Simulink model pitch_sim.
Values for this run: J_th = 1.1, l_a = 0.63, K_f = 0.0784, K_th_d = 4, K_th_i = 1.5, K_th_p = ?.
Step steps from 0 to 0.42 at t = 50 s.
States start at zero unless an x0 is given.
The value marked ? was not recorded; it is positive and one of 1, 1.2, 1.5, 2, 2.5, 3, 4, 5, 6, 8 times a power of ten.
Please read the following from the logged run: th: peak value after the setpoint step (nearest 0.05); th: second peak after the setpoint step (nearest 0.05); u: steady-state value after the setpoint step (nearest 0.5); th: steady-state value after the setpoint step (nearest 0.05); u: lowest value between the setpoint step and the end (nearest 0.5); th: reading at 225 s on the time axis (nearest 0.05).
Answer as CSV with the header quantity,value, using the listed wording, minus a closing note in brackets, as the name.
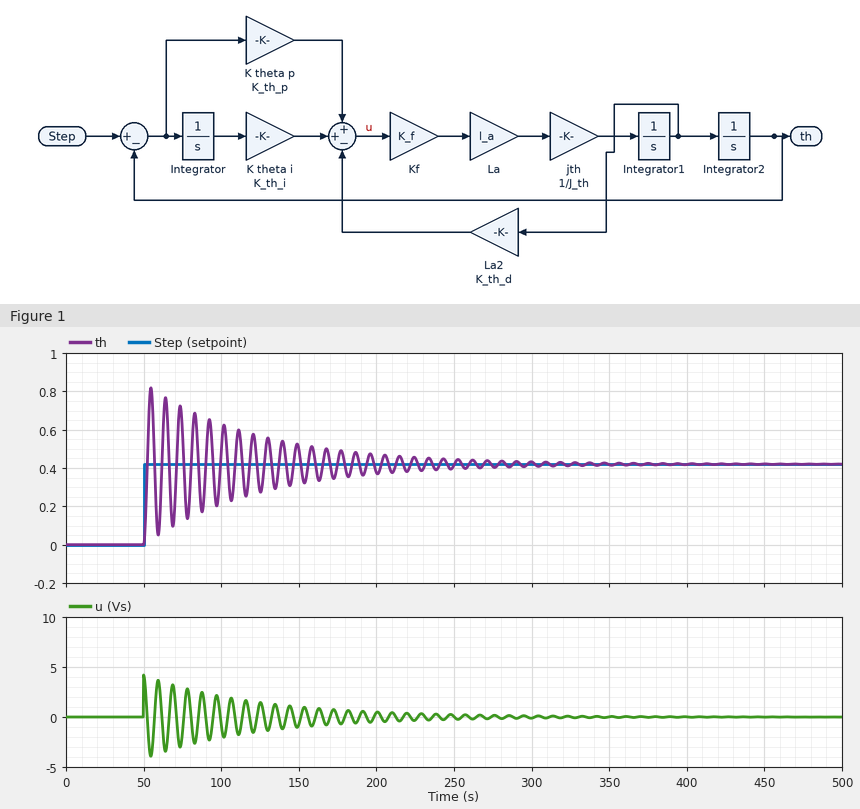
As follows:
quantity,value
th: peak value after the setpoint step,0.80
th: second peak after the setpoint step,0.75
u: steady-state value after the setpoint step,0.0
th: steady-state value after the setpoint step,0.40
u: lowest value between the setpoint step and the end,-4.0
th: reading at 225 s on the time axis,0.45
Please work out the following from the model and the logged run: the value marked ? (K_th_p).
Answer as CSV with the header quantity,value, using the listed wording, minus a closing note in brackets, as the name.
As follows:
quantity,value
the value marked ?,10
